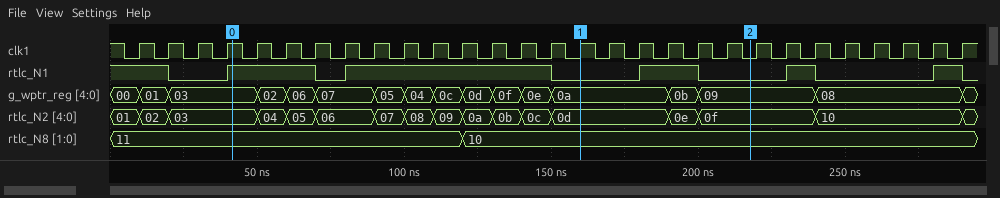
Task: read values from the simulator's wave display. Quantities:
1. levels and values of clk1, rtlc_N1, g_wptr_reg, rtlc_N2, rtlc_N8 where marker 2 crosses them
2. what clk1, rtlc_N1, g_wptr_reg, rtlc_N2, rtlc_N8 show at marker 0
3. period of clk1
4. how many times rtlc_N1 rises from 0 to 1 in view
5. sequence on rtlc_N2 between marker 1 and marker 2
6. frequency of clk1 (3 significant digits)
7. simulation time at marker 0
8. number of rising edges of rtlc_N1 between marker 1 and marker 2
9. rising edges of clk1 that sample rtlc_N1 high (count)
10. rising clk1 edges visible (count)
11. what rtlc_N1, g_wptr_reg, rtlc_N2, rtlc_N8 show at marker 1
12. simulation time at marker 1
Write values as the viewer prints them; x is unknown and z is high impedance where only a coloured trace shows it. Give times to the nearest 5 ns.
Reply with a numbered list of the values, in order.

1. clk1=0, rtlc_N1=0, g_wptr_reg=09, rtlc_N2=0f, rtlc_N8=10
2. clk1=1, rtlc_N1=1, g_wptr_reg=03, rtlc_N2=03, rtlc_N8=11
3. 10 ns
4. 5
5. 0d, 0e, 0f
6. 100 MHz
7. 40 ns
8. 1
9. 16
10. 29
11. rtlc_N1=0, g_wptr_reg=0a, rtlc_N2=0d, rtlc_N8=10
12. 160 ns
